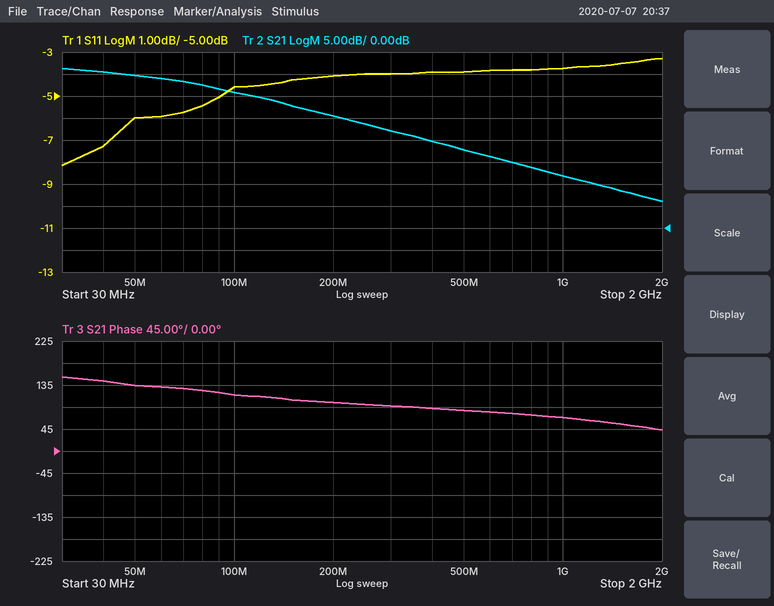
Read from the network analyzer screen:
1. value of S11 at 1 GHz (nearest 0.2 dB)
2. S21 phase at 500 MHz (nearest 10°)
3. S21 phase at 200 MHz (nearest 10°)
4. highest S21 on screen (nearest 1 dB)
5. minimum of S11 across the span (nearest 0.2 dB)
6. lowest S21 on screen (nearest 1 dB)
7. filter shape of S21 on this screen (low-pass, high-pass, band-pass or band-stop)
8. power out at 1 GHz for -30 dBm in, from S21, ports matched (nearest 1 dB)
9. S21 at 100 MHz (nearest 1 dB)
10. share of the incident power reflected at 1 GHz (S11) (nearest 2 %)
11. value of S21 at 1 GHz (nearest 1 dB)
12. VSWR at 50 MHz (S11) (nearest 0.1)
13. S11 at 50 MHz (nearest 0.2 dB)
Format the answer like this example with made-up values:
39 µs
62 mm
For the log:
-3.8 dB
80°
100°
36 dB
-8.2 dB
6 dB
low-pass
-18 dBm
31 dB
42 %
12 dB
3.0
-6.0 dB
